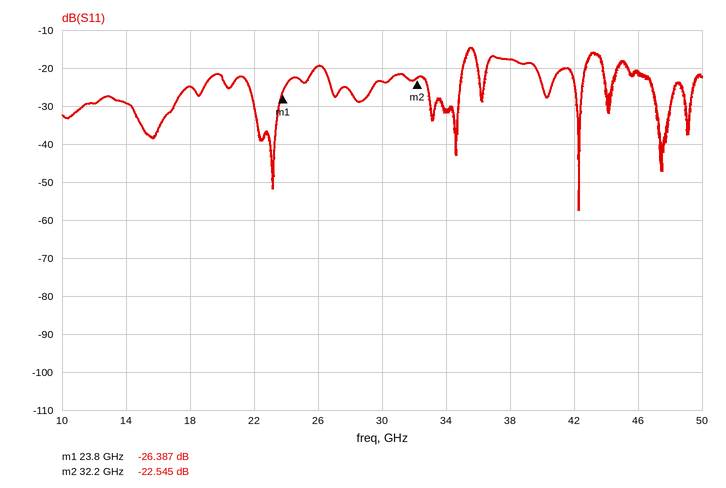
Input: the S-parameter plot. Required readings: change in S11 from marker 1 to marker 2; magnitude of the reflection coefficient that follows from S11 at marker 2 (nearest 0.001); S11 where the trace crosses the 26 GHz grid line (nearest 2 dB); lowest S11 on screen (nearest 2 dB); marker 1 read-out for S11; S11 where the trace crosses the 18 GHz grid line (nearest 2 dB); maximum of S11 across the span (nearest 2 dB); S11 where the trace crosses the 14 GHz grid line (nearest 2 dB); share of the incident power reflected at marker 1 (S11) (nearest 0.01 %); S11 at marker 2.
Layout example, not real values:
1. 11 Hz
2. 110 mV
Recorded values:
1. 3.842 dB
2. 0.075
3. -20 dB
4. -58 dB
5. -26.387 dB
6. -24 dB
7. -14 dB
8. -30 dB
9. 0.23 %
10. -22.545 dB
